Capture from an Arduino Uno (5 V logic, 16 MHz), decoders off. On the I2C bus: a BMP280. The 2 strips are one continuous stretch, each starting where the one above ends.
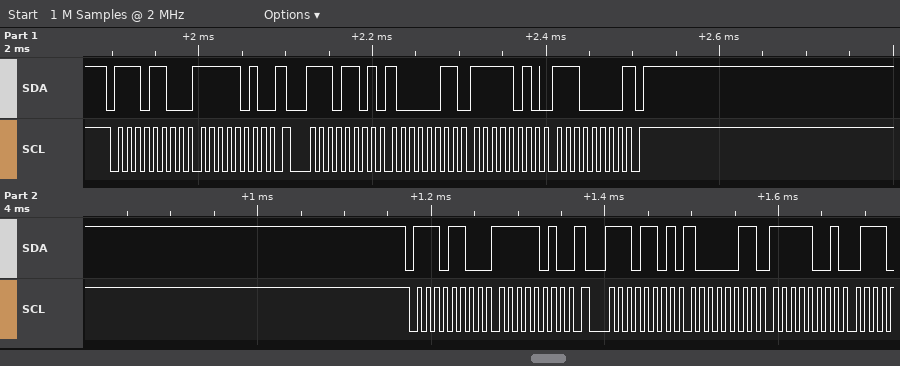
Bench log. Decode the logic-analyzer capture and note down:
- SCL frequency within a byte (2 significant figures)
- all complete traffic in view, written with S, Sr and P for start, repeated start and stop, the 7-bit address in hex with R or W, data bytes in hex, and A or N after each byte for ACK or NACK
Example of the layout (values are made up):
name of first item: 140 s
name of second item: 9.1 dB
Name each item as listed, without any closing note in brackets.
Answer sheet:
SCL frequency within a byte: 100 kHz
all complete traffic in view, written with S, Sr and P for start, repeated start and stop, the 7-bit address in hex with R or W, data bytes in hex, and A or N after each byte for ACK or NACK: S 76W A FA A Sr 76R A 83 A FA A E0 N P S 76W A FA A Sr 76R A 83 A F9 A
